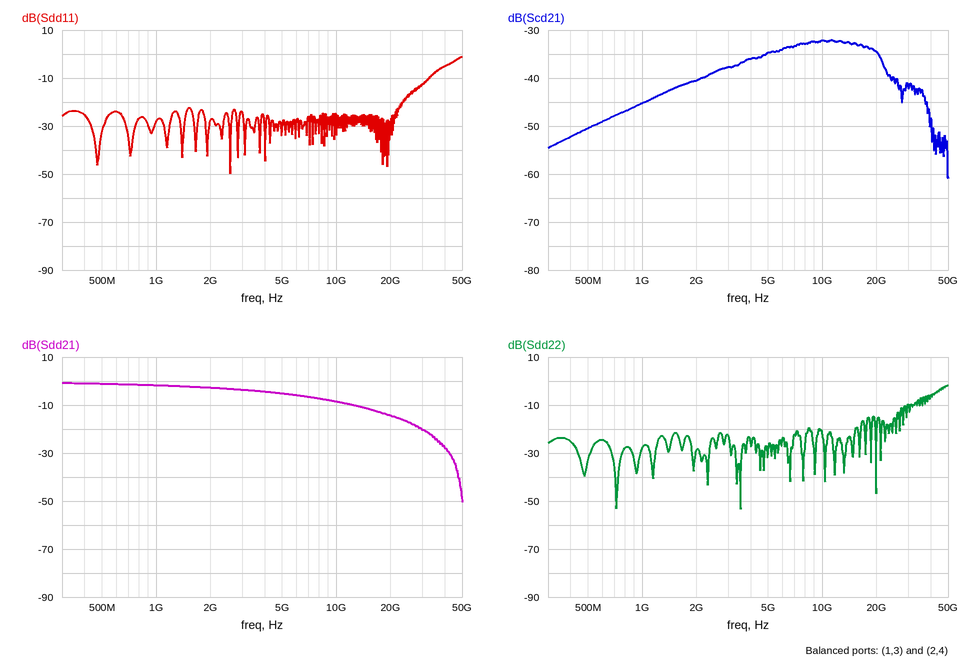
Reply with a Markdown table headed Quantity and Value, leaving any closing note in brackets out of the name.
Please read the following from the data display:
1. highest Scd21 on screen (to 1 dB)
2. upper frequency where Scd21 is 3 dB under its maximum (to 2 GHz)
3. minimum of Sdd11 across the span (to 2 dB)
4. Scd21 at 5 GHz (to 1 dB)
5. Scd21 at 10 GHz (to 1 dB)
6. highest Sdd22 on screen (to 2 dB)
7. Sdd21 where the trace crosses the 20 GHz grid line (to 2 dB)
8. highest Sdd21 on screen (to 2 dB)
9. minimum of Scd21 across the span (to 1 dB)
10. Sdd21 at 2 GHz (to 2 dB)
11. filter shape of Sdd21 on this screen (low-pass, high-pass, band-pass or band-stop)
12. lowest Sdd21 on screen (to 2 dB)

| Quantity | Value |
|---|---|
| highest Scd21 on screen | -32 dB |
| upper frequency where Scd21 is 3 dB under its maximum | 20 GHz |
| minimum of Sdd11 across the span | -50 dB |
| Scd21 at 5 GHz | -35 dB |
| Scd21 at 10 GHz | -32 dB |
| highest Sdd22 on screen | -2 dB |
| Sdd21 where the trace crosses the 20 GHz grid line | -14 dB |
| highest Sdd21 on screen | 0 dB |
| minimum of Scd21 across the span | -61 dB |
| Sdd21 at 2 GHz | -2 dB |
| filter shape of Sdd21 on this screen | low-pass |
| lowest Sdd21 on screen | -50 dB |
